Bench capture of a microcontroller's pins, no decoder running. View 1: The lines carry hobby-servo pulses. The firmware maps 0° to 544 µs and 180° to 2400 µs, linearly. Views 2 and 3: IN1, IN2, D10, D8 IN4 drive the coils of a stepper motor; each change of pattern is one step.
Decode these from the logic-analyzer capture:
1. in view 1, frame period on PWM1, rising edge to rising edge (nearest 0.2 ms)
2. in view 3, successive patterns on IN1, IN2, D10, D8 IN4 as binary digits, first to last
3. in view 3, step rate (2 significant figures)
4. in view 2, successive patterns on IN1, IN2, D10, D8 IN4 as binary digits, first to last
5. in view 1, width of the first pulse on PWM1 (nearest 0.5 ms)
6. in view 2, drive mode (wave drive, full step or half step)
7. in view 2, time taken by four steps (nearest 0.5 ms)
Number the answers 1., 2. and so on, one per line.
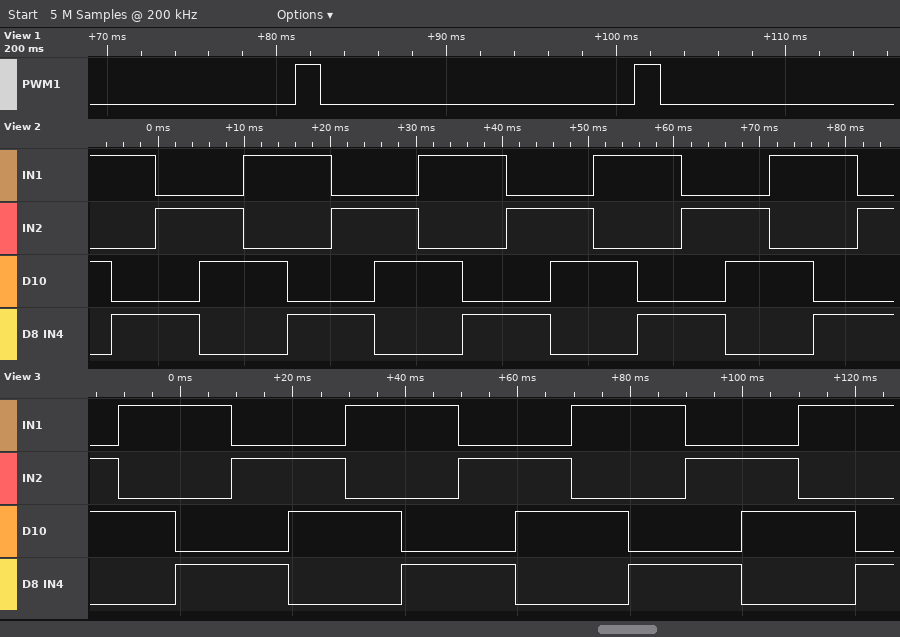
1. 20.0 ms
2. 0110 1010 1001 0101 0110 1010 1001 0101 0110 1010 1001 0101 0110 1010 1001
3. 99 steps/s
4. 1010 1001 0101 0110 1010 1001 0101 0110 1010 1001 0101 0110 1010 1001 0101 0110 1010 1001 0101
5. 1.5 ms
6. full step
7. 20.5 ms
